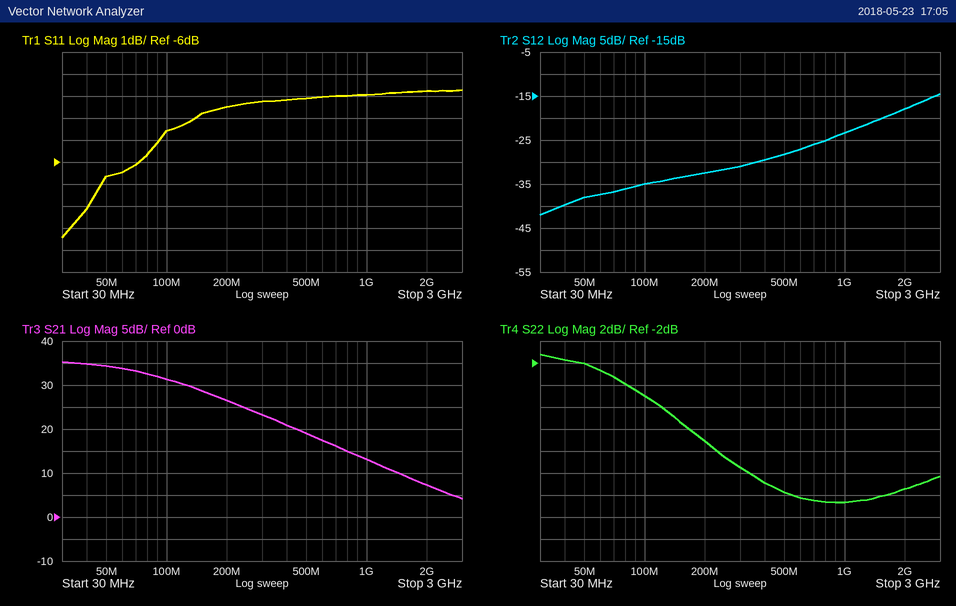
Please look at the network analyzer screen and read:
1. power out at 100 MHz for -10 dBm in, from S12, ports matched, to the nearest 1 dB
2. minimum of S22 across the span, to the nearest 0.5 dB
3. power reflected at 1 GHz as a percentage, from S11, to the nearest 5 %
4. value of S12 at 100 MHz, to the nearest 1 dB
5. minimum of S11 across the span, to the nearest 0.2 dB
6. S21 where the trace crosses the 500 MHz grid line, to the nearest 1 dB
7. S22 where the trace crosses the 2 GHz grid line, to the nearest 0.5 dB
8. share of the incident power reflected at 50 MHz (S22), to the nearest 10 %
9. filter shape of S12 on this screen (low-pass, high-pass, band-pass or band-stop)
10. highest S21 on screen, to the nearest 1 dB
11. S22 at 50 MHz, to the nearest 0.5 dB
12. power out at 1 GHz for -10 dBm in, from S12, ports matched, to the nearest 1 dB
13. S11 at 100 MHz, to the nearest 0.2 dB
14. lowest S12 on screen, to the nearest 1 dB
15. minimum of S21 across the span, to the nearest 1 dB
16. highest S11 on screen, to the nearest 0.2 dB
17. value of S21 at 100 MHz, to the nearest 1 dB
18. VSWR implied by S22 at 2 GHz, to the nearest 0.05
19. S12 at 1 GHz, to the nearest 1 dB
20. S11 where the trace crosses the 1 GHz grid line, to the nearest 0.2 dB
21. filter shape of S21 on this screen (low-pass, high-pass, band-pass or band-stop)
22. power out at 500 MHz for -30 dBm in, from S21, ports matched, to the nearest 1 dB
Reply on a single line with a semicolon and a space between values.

-45 dBm; -14.5 dB; 50 %; -35 dB; -9.4 dB; 19 dB; -13.5 dB; 60 %; high-pass; 35 dB; -2.0 dB; -33 dBm; -4.6 dB; -42 dB; 4 dB; -2.8 dB; 31 dB; 1.55; -23 dB; -3.0 dB; low-pass; -11 dBm
